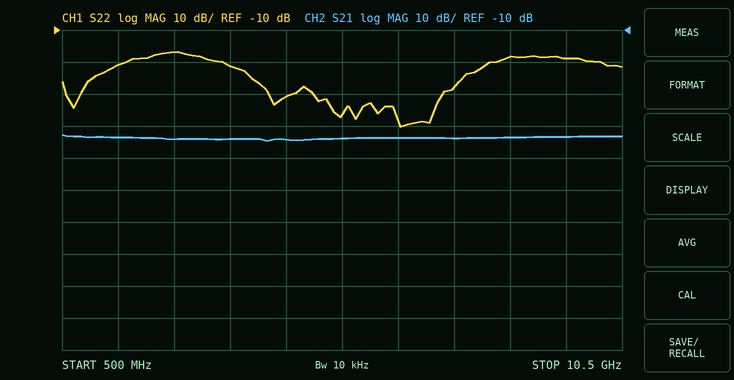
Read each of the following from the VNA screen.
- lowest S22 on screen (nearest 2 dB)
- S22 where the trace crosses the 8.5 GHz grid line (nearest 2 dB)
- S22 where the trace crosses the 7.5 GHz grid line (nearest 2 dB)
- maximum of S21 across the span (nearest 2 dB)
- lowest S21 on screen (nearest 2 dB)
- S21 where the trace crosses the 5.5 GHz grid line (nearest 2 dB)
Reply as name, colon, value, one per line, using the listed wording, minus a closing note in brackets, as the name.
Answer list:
lowest S22 on screen: -40 dB
S22 where the trace crosses the 8.5 GHz grid line: -18 dB
S22 where the trace crosses the 7.5 GHz grid line: -28 dB
maximum of S21 across the span: -42 dB
lowest S21 on screen: -44 dB
S21 where the trace crosses the 5.5 GHz grid line: -44 dB
